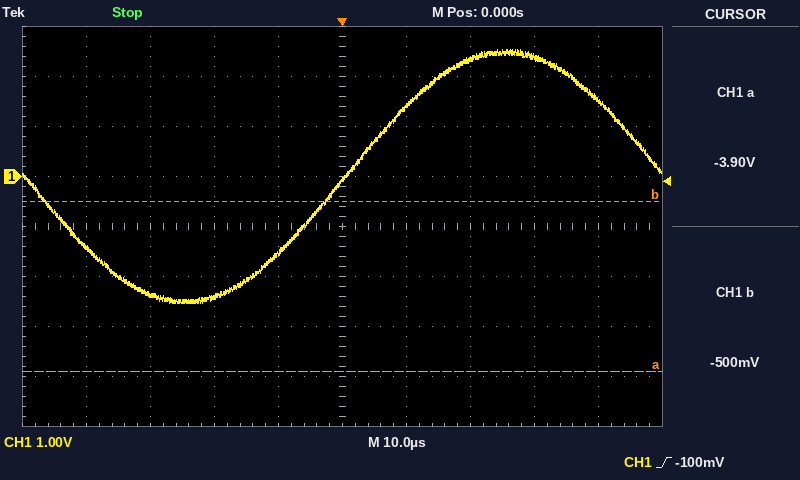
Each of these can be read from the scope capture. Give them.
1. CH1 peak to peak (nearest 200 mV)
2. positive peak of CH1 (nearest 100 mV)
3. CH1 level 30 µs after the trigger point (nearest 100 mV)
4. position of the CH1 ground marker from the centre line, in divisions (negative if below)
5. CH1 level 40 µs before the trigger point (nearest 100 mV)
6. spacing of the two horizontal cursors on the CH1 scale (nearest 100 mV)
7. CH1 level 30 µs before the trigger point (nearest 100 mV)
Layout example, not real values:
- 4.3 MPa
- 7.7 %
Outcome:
- 5.0 V
- 2.5 V
- 2.4 V
- +1.0 div
- -1.4 V
- 3.4 V
- -2.4 V
